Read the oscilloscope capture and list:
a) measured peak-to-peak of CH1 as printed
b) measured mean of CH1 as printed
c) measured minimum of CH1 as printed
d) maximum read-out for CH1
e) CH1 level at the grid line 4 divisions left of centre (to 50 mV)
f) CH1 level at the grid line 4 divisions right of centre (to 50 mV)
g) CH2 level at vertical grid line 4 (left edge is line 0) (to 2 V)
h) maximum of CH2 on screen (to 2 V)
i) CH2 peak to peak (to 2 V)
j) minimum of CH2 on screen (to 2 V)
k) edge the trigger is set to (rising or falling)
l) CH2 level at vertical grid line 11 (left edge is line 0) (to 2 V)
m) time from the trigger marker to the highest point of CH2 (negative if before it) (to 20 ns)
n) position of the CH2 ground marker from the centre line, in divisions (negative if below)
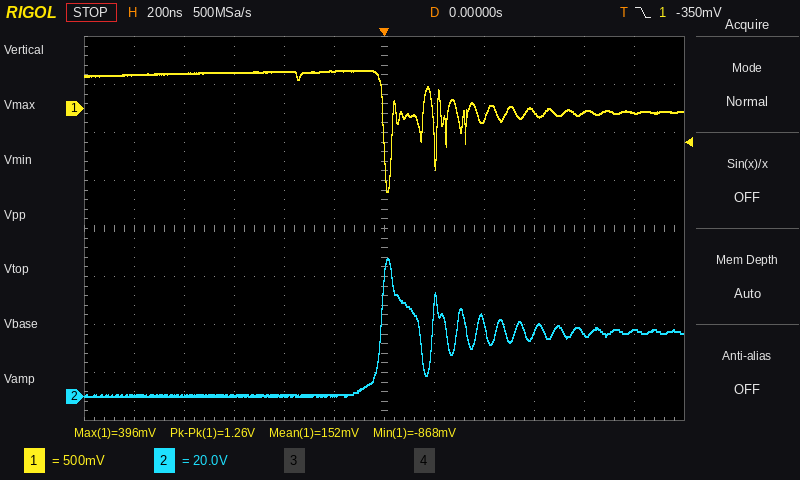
1.26 V
152 mV
-868 mV
396 mV
350 mV
-50 mV
0 V
58 V
58 V
0 V
falling
28 V
+20 ns
-3.5 div
